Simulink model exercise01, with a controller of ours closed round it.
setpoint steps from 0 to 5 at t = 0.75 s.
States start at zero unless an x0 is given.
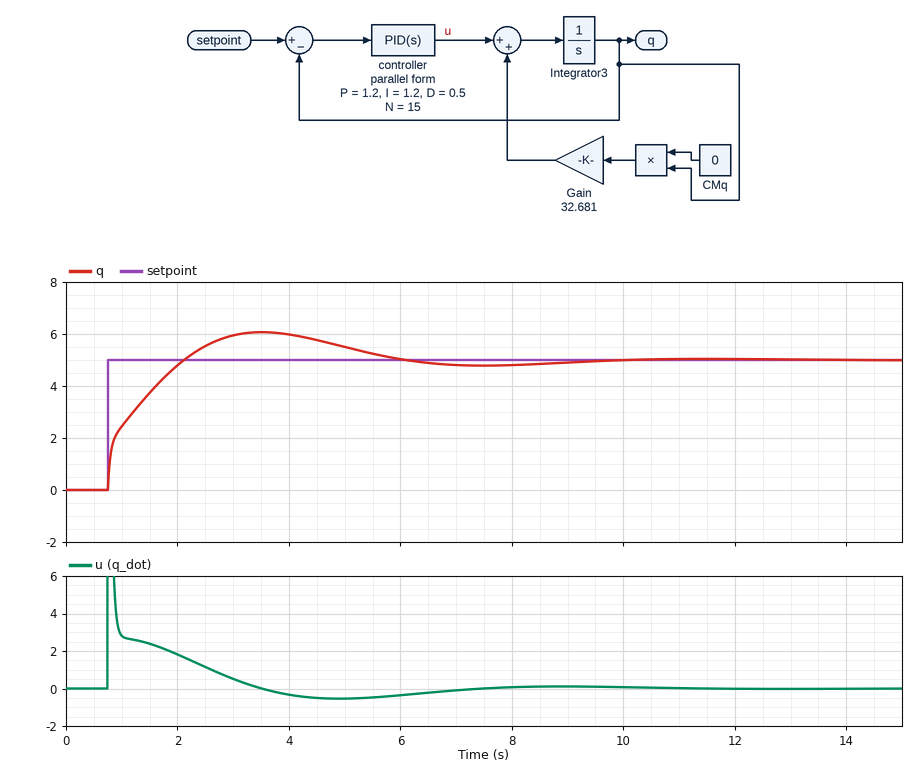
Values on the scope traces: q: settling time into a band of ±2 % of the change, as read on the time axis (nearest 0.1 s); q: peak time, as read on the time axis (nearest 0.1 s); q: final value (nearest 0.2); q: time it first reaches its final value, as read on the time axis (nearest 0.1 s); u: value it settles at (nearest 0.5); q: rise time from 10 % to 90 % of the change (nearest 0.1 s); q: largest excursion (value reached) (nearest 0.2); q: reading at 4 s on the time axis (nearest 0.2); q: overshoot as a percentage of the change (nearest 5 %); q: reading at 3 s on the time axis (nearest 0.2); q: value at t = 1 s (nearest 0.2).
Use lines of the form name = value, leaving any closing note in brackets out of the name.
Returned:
q: settling time into a band of ±2 % of the change, as read on the time axis = 9.0 s
q: peak time, as read on the time axis = 3.5 s
q: final value = 5.0
q: time it first reaches its final value, as read on the time axis = 2.1 s
u: value it settles at = 0.0
q: rise time from 10 % to 90 % of the change = 1.1 s
q: largest excursion (value reached) = 6.0
q: reading at 4 s on the time axis = 6.0
q: overshoot as a percentage of the change = 20 %
q: reading at 3 s on the time axis = 6.0
q: value at t = 1 s = 2.4
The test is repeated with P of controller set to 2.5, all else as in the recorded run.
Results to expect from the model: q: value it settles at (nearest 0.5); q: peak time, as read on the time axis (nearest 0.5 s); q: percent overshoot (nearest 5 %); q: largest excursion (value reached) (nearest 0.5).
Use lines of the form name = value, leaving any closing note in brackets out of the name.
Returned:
q: value it settles at = 5.0
q: peak time, as read on the time axis = 3.0 s
q: percent overshoot = 10 %
q: largest excursion (value reached) = 5.5
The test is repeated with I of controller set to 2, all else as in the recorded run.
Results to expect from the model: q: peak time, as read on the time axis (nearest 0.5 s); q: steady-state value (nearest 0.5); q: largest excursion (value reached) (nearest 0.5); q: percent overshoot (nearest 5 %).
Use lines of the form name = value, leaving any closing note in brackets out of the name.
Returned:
q: peak time, as read on the time axis = 3.0 s
q: steady-state value = 5.0
q: largest excursion (value reached) = 6.5
q: percent overshoot = 25 %
